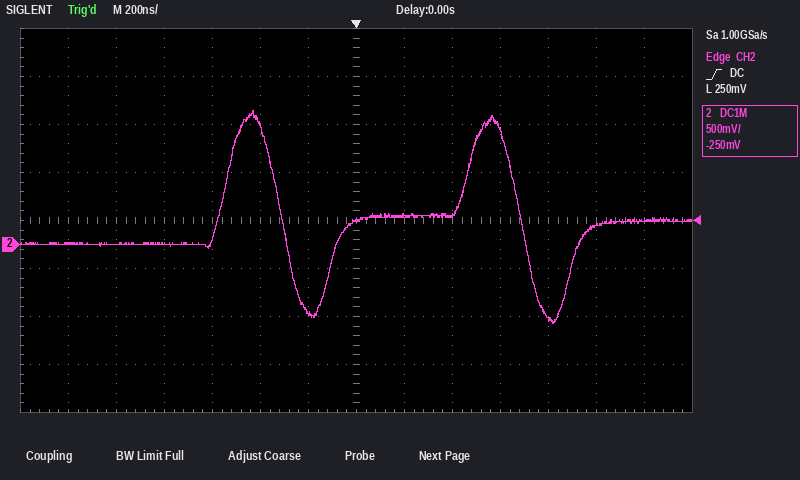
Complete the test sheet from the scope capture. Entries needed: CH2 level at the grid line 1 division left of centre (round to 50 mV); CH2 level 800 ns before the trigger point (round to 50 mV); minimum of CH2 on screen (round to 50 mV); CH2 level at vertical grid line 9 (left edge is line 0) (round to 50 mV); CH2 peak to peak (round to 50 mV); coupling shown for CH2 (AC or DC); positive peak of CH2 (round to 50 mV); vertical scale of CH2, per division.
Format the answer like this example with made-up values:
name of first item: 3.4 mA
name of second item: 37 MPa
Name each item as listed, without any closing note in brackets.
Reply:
CH2 level at the grid line 1 division left of centre: -700 mV
CH2 level 800 ns before the trigger point: 0 mV
minimum of CH2 on screen: -800 mV
CH2 level at vertical grid line 9 (left edge is line 0): 300 mV
CH2 peak to peak: 2.20 V
coupling shown for CH2: DC
positive peak of CH2: 1.40 V
vertical scale of CH2, per division: 500 mV
